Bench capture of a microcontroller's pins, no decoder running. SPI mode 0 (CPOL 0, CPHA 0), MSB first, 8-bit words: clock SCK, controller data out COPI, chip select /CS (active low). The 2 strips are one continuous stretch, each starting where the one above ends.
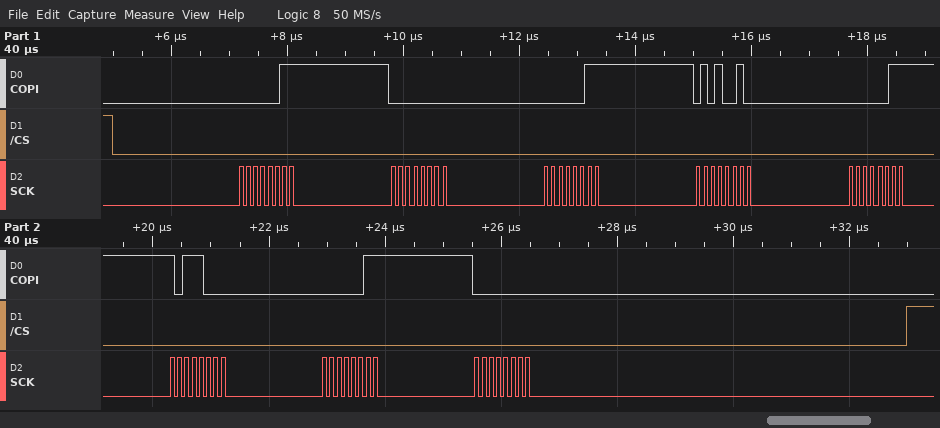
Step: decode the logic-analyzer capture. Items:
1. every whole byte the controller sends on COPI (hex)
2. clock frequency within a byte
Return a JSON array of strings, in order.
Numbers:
["03 00 03 52 03 B8 03 00", "8 MHz"]
